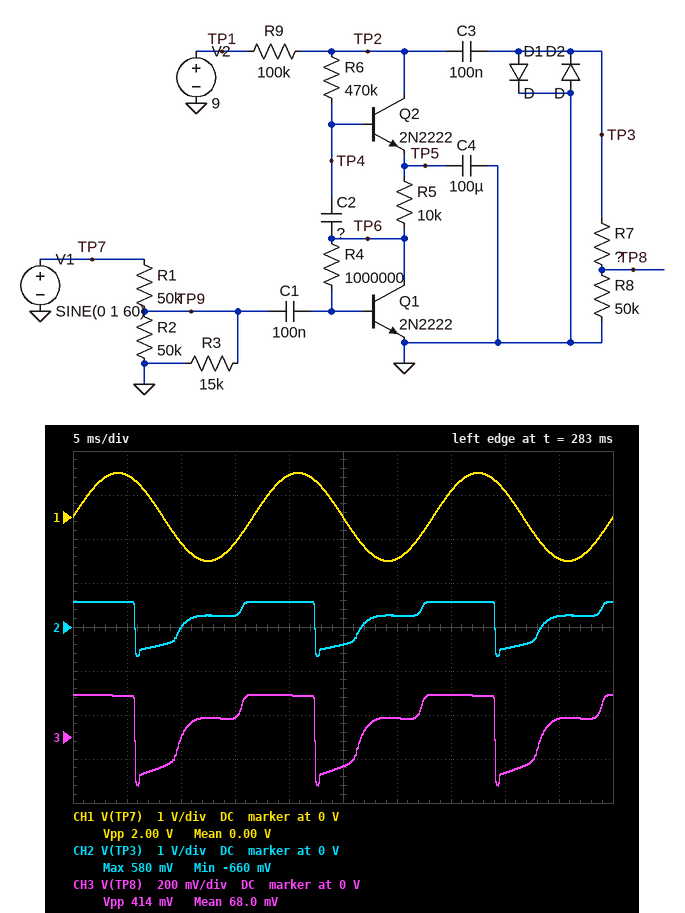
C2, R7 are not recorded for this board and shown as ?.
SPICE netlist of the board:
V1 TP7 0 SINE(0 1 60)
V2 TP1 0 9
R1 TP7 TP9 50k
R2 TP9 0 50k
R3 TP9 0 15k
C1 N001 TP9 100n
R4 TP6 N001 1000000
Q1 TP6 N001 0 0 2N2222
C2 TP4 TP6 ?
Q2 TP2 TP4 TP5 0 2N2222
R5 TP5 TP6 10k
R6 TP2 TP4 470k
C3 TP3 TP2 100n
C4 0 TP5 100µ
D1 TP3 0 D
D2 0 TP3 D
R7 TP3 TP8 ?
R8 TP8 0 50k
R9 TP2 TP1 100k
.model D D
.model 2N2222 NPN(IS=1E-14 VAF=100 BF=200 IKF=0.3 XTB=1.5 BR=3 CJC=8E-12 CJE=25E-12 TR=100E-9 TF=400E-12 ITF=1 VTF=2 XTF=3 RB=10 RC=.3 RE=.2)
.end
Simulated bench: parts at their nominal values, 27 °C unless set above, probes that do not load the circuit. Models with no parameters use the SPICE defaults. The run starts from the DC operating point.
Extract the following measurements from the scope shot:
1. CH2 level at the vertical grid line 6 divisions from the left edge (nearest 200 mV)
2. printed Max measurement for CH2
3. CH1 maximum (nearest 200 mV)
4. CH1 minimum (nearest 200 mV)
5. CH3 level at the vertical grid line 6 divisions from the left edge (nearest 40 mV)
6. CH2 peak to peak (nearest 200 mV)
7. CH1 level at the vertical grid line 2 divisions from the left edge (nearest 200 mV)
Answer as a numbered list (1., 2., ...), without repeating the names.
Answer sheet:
1. 200 mV
2. 580 mV
3. 1.0 V
4. -1.0 V
5. 80 mV
6. 1.2 V
7. -600 mV
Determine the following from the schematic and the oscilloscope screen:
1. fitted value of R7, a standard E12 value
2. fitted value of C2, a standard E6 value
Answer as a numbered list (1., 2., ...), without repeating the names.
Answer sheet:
1. 100 kΩ
2. 68 nF
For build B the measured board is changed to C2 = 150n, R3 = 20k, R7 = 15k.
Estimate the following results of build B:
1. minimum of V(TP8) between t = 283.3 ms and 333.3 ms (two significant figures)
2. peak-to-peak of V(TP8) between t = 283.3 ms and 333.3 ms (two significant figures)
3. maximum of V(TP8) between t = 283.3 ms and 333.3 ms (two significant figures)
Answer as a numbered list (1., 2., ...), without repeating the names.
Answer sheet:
1. -500 mV
2. 950 mV
3. 440 mV
